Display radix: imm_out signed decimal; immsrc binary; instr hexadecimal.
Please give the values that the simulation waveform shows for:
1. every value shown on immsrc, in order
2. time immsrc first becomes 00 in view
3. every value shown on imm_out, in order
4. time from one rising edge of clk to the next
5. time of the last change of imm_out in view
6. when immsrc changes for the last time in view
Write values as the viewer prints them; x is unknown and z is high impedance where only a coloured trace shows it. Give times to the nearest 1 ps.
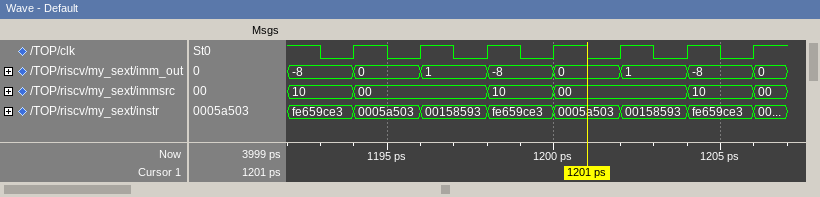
10, 00, 10, 00, 10, 00
1194 ps
-8, 0, 1, -8, 0, 1, -8, 0
2 ps
1206 ps
1206 ps
